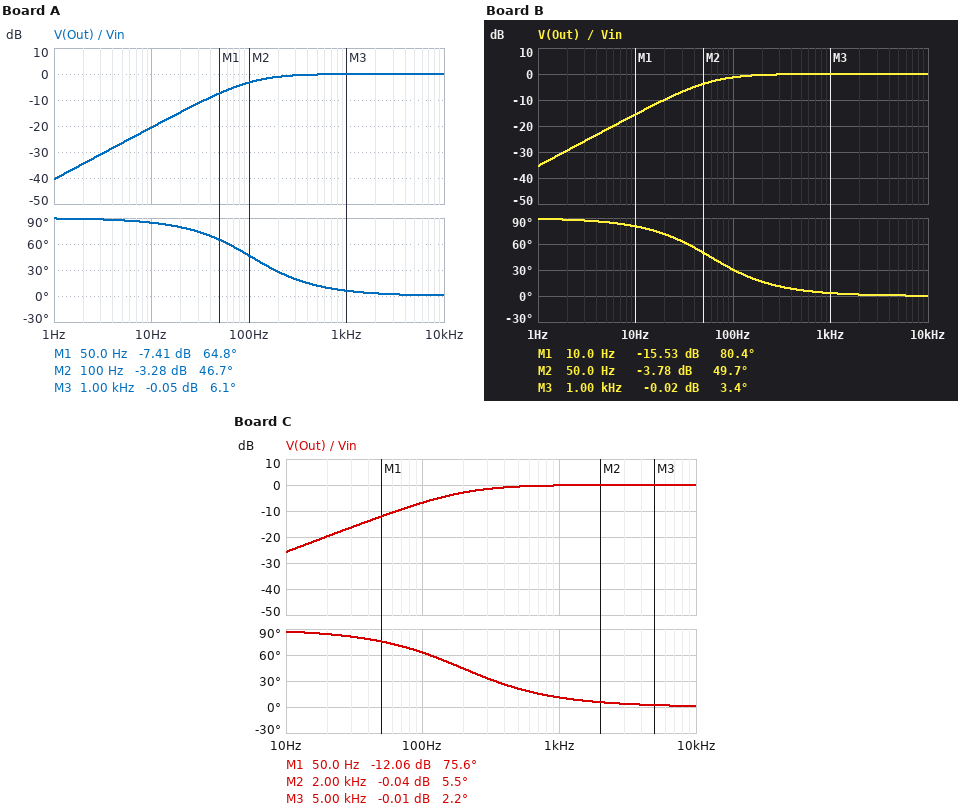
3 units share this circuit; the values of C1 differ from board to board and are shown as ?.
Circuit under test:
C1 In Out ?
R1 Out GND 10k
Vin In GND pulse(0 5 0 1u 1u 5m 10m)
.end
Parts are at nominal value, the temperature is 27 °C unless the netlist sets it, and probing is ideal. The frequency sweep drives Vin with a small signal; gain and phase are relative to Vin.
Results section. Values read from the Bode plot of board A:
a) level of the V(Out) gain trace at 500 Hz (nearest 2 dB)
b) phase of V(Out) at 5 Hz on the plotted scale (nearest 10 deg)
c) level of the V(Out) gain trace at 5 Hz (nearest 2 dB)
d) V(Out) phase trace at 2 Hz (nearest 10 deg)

0 dB
90 deg
-26 dB
90 deg
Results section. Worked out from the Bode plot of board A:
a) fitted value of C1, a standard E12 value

150 nF
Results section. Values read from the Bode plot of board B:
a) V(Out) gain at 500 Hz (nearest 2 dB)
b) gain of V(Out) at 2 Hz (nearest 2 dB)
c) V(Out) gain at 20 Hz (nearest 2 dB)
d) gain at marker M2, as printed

0 dB
-30 dB
-10 dB
-3.78 dB
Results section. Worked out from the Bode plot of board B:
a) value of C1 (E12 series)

270 nF
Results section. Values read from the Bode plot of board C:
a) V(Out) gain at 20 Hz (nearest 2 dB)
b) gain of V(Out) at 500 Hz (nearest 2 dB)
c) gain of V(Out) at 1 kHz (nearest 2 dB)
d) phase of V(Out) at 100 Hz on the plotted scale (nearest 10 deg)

-20 dB
0 dB
0 dB
60 deg
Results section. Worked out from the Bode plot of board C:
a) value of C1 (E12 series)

82 nF
